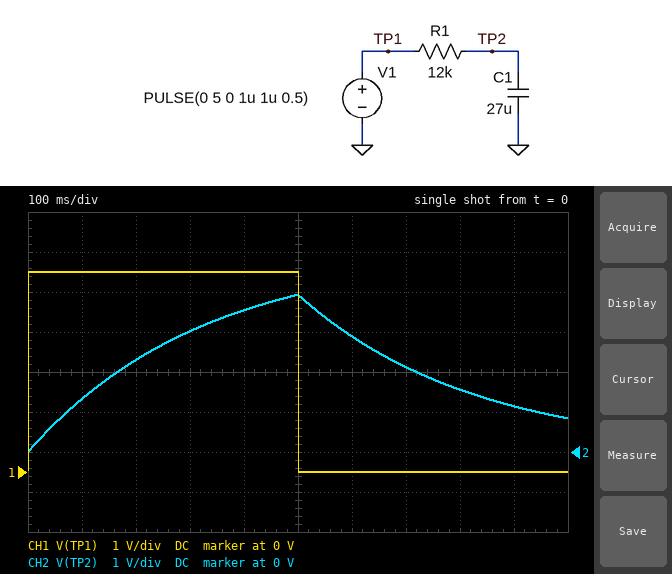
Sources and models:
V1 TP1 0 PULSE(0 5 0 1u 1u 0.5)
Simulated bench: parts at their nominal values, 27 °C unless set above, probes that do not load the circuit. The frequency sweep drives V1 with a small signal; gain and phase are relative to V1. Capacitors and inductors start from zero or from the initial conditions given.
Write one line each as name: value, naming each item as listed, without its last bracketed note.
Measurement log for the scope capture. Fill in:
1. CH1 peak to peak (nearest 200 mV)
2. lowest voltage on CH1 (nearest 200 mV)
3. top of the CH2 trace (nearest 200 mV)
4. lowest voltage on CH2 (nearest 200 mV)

CH1 peak to peak: 5.0 V
lowest voltage on CH1: 0 V
top of the CH2 trace: 4.0 V
lowest voltage on CH2: 0 V
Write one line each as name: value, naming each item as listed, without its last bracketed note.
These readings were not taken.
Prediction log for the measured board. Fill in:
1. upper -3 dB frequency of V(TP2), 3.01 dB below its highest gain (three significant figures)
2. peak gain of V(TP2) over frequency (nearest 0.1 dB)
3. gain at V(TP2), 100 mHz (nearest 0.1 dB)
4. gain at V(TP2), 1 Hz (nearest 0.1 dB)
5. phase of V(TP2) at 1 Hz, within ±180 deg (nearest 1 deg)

upper -3 dB frequency of V(TP2), 3.01 dB below its highest gain: 491 mHz
peak gain of V(TP2) over frequency: 0 dB
gain at V(TP2), 100 mHz: -0.2 dB
gain at V(TP2), 1 Hz: -7.1 dB
phase of V(TP2) at 1 Hz, within ±180 deg: -64 deg
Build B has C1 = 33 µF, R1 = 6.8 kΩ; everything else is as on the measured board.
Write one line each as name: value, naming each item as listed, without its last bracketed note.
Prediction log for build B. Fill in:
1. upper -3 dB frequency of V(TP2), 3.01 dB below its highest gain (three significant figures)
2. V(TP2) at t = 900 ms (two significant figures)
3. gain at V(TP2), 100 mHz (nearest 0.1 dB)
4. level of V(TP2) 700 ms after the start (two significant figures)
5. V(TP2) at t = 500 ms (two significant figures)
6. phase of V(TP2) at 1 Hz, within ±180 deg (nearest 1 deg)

upper -3 dB frequency of V(TP2), 3.01 dB below its highest gain: 709 mHz
V(TP2) at t = 900 ms: 750 mV
gain at V(TP2), 100 mHz: -0.1 dB
level of V(TP2) 700 ms after the start: 1.8 V
V(TP2) at t = 500 ms: 4.5 V
phase of V(TP2) at 1 Hz, within ±180 deg: -55 deg
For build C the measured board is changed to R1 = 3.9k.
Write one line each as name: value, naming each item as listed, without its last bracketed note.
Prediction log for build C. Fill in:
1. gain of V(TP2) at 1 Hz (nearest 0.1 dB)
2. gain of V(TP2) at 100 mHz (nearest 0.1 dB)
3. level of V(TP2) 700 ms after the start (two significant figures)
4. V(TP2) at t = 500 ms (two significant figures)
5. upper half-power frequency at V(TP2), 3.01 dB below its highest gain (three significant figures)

gain of V(TP2) at 1 Hz: -1.6 dB
gain of V(TP2) at 100 mHz: 0 dB
level of V(TP2) 700 ms after the start: 740 mV
V(TP2) at t = 500 ms: 5.0 V
upper half-power frequency at V(TP2), 3.01 dB below its highest gain: 1.51 Hz
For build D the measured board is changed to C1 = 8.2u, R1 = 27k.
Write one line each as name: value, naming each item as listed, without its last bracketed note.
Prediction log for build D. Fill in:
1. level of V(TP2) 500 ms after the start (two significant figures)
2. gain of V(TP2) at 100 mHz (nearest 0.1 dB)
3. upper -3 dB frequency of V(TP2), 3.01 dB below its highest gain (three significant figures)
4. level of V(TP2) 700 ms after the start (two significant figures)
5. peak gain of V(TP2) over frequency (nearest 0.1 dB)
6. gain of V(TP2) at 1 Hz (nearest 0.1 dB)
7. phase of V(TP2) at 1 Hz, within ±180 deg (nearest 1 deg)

level of V(TP2) 500 ms after the start: 4.5 V
gain of V(TP2) at 100 mHz: -0.1 dB
upper -3 dB frequency of V(TP2), 3.01 dB below its highest gain: 719 mHz
level of V(TP2) 700 ms after the start: 1.8 V
peak gain of V(TP2) over frequency: 0 dB
gain of V(TP2) at 1 Hz: -4.7 dB
phase of V(TP2) at 1 Hz, within ±180 deg: -54 deg
